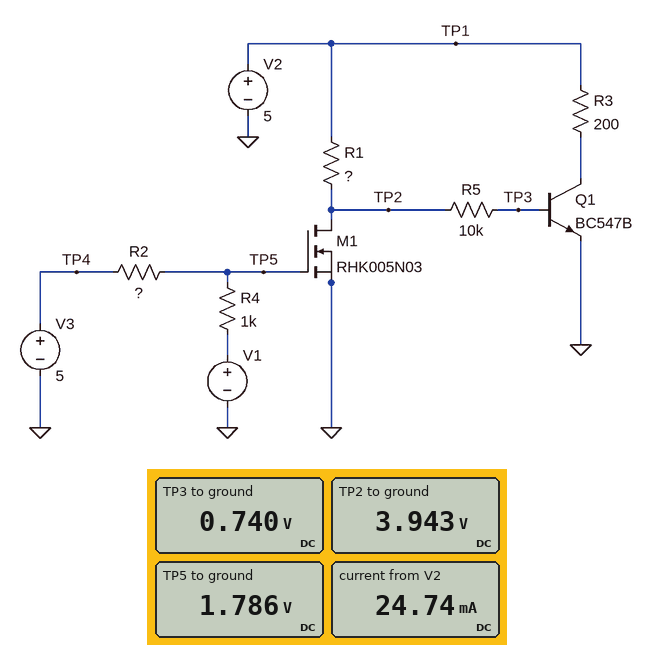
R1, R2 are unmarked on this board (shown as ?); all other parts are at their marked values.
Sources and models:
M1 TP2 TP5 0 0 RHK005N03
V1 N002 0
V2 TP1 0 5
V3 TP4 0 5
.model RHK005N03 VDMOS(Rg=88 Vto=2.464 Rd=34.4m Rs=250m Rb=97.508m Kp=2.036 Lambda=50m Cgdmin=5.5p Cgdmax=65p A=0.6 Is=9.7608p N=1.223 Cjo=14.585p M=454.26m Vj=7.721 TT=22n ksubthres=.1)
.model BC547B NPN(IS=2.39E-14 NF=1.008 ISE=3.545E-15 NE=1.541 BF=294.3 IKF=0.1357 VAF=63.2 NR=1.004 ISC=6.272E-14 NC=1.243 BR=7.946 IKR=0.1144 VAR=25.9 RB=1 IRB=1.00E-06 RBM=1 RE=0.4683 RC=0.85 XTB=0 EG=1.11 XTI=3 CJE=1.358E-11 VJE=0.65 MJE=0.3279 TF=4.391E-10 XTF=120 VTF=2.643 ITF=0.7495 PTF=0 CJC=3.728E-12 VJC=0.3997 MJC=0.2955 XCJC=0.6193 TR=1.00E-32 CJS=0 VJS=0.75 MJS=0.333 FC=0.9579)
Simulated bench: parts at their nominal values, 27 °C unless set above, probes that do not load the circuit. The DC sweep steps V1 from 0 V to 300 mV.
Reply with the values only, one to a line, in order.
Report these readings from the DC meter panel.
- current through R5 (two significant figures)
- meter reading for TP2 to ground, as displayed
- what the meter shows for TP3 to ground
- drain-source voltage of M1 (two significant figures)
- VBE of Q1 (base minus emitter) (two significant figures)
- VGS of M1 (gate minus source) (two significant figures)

320 µA
3.943 V
0.740 V
3.9 V
740 mV
1.8 V
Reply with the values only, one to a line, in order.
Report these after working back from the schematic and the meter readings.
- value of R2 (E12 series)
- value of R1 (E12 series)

1.8 kΩ
3.3 kΩ
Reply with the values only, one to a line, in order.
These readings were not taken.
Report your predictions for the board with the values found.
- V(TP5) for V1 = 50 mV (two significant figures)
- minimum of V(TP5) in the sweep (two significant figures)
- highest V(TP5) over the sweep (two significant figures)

1.8 V
1.8 V
2.0 V
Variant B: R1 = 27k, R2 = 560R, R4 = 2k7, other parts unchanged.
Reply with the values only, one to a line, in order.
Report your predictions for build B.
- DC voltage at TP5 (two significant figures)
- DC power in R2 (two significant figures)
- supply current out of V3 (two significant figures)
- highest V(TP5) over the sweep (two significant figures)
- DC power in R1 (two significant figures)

4.1 V
1.3 mW
1.5 mA
4.2 V
930 µW
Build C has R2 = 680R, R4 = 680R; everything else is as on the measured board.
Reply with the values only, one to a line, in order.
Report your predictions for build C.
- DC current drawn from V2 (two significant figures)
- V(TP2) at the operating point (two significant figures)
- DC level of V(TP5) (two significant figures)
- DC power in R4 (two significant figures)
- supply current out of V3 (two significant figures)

1.5 mA
9.2 mV
2.5 V
9.2 mW
3.7 mA
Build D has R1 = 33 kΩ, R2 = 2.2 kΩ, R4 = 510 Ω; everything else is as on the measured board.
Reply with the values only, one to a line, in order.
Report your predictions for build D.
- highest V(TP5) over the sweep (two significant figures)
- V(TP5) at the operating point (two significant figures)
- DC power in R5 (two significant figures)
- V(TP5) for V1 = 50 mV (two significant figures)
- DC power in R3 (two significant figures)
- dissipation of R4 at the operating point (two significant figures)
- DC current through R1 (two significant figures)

1.2 V
940 mV
98 µW
980 mV
110 mW
1.7 mW
99 µA
